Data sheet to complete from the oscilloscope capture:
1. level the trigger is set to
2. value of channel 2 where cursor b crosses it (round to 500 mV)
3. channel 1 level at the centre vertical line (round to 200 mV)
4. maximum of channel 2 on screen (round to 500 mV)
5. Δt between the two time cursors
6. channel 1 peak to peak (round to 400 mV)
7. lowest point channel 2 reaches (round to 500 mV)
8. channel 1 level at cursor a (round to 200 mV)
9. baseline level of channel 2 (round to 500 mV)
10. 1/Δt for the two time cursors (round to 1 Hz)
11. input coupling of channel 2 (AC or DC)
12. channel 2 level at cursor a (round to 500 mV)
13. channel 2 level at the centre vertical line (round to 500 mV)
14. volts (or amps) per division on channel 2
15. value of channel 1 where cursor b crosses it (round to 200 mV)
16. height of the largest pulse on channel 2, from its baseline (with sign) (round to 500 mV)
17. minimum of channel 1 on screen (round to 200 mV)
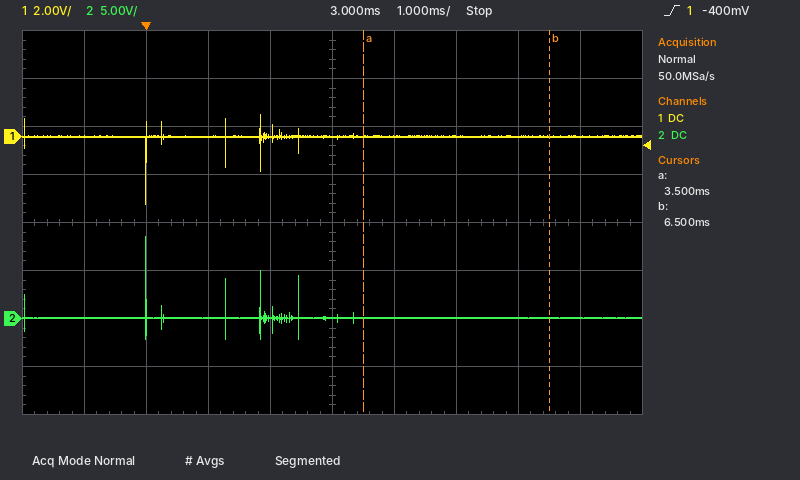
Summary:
-400 mV
0.0 V
0.0 V
8.5 V
3.0 ms
3.6 V
-2.0 V
0.0 V
0.0 V
333 Hz
DC
0.0 V
0.0 V
5 V
0.0 V
+8.5 V
-2.8 V
